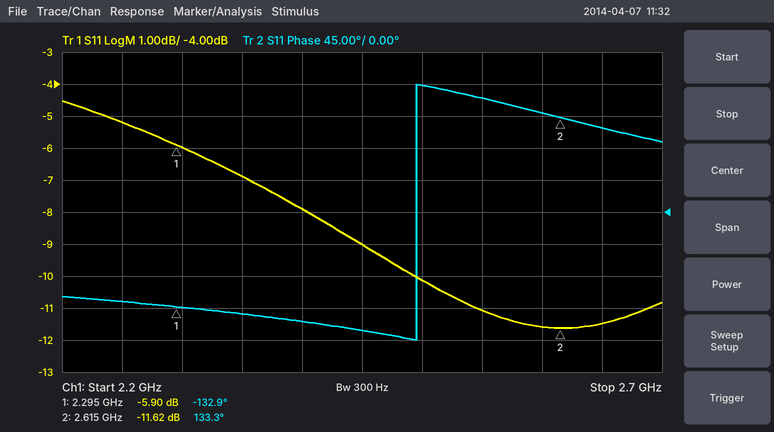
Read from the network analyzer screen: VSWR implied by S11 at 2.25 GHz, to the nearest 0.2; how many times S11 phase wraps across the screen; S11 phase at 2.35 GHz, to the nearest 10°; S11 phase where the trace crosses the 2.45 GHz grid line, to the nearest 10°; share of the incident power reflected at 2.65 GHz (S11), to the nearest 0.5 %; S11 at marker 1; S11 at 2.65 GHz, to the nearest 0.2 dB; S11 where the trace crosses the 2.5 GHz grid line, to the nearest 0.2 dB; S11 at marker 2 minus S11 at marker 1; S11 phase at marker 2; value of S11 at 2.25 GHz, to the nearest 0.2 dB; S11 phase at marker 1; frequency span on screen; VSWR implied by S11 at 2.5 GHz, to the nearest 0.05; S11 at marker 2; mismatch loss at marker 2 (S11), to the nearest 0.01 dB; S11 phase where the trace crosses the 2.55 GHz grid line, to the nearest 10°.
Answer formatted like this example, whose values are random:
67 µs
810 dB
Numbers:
3.4
1
-140°
-170°
7.0 %
-5.90 dB
-11.4 dB
-10.2 dB
-5.72 dB
133.3°
-5.2 dB
-132.9°
500 MHz
1.90
-11.62 dB
0.31 dB
160°
